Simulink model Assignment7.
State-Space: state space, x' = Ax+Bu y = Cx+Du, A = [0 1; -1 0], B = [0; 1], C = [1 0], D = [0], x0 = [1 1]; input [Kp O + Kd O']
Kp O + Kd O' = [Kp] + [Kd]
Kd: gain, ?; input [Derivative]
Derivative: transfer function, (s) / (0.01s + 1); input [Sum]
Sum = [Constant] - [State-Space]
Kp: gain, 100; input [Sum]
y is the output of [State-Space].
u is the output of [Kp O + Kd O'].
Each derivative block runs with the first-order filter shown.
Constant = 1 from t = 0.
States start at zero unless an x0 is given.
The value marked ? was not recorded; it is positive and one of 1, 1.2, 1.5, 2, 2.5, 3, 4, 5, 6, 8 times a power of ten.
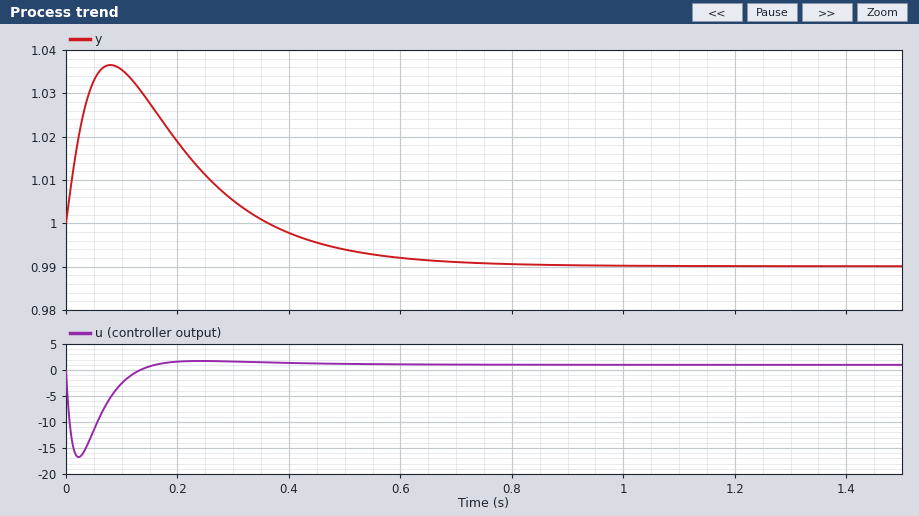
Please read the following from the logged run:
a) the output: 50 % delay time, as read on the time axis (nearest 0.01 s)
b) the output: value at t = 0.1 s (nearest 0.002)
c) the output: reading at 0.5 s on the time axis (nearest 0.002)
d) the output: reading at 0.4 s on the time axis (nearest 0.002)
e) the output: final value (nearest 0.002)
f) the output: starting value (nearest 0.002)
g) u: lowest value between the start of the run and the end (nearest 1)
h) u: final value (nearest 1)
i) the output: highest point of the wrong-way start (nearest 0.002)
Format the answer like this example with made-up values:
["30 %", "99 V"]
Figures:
["0.46 s", "1.036", "0.994", "0.998", "0.990", "1.000", "-17", "1", "1.036"]
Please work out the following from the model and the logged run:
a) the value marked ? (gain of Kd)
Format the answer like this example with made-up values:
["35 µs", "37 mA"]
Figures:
["20"]
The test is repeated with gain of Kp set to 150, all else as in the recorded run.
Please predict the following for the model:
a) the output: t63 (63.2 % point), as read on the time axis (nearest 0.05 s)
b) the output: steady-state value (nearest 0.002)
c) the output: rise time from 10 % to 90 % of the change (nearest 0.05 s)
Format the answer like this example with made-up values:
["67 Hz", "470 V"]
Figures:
["0.35 s", "0.994", "0.15 s"]
